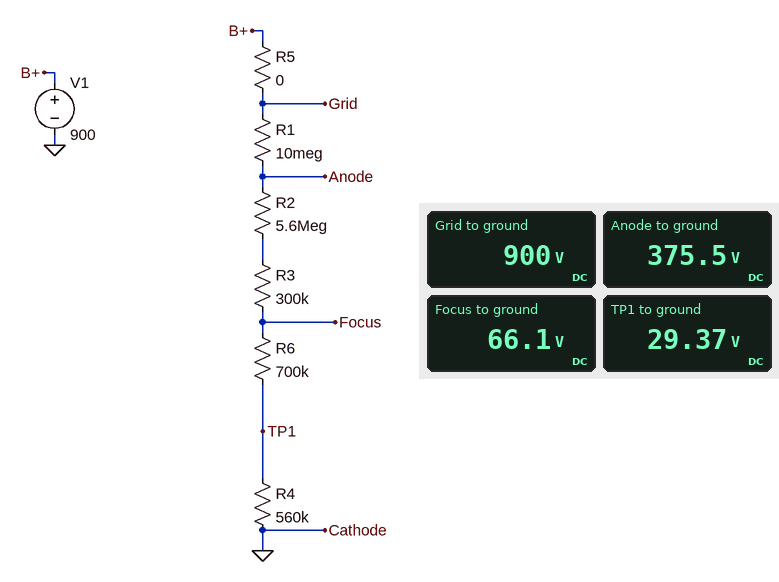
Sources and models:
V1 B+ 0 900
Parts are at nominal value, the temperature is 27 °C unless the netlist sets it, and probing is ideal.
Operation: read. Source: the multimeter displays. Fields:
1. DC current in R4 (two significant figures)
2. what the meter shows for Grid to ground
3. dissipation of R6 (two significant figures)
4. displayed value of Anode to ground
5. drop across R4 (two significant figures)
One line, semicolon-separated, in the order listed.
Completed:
52 µA; 900 V; 1.9 mW; 375.5 V; 29 V
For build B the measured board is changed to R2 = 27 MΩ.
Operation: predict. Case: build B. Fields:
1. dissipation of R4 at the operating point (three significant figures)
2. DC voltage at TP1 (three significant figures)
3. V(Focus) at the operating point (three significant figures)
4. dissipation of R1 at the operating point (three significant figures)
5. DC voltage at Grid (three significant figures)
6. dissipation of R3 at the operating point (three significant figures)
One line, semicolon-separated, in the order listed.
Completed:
305 µW; 13.1 V; 29.4 V; 5.45 mW; 900 V; 163 µW
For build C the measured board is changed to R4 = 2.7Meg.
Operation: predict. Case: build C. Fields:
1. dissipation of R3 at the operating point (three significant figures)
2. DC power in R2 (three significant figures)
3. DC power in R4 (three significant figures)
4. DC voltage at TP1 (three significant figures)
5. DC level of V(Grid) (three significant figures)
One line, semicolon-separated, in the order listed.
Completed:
652 µW; 12.2 mW; 5.87 mW; 126 V; 900 V
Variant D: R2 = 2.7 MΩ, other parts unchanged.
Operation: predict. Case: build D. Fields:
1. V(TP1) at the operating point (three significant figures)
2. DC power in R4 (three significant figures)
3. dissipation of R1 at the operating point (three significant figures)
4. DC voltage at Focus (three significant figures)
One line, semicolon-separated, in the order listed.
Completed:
35.3 V; 2.23 mW; 39.8 mW; 79.5 V
